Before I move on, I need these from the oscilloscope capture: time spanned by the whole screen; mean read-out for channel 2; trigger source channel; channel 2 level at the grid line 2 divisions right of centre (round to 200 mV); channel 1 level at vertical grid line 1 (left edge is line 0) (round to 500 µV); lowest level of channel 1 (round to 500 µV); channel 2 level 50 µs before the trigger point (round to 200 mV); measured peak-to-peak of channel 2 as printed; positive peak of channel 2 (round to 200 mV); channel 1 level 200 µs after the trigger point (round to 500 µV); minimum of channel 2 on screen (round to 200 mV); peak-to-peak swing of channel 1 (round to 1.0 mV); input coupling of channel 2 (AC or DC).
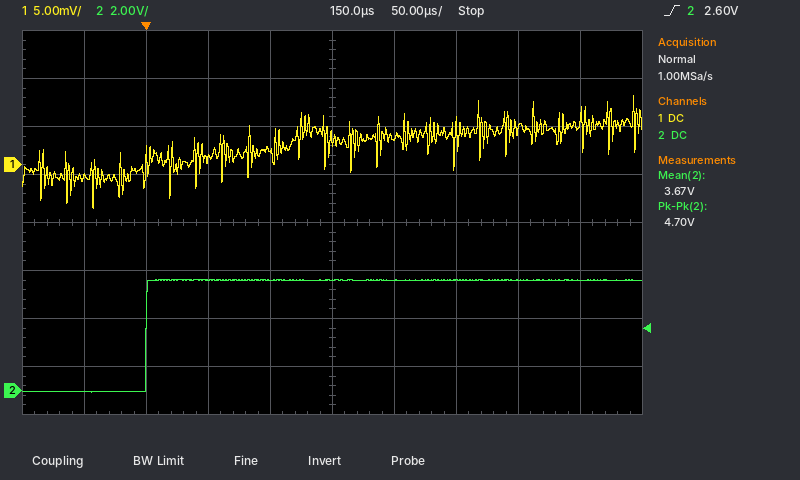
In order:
500 µs
3.67 V
channel 2
4.6 V
-1.5 mV
-4.5 mV
0.0 V
4.70 V
4.6 V
3.0 mV
0.0 V
12.0 mV
DC
